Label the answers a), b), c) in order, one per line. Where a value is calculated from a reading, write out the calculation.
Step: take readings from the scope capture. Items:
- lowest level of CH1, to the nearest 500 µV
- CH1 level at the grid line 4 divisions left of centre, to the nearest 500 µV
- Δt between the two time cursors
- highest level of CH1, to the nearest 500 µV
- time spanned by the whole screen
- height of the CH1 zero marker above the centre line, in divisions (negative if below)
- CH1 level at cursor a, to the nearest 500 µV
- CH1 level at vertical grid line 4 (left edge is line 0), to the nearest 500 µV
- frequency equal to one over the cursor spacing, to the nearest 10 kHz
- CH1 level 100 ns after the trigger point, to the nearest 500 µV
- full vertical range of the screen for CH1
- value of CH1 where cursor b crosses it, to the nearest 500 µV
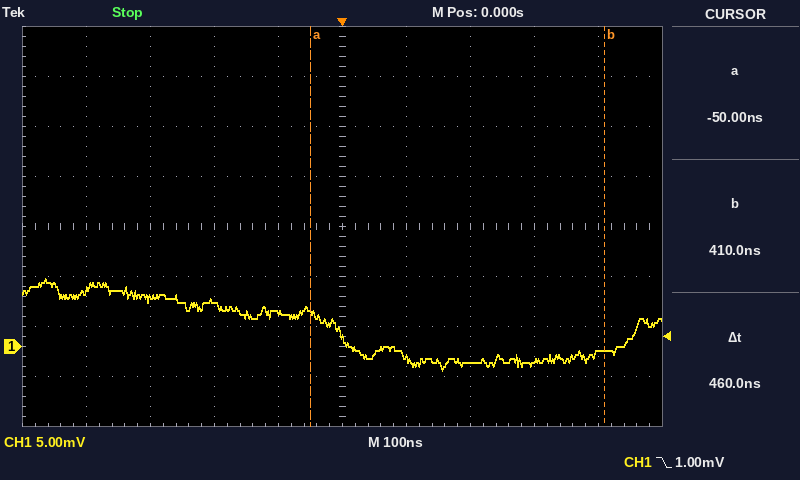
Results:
a) -2.5 mV
b) 5.5 mV
c) 460 ns
d) 7.0 mV
e) 1 µs
f) -2.4 div
g) 3.5 mV
h) 3.5 mV
i) 1 / 460 ns ≈ 2.17 MHz
j) -1.0 mV
k) 40 mV
l) -500 µV
